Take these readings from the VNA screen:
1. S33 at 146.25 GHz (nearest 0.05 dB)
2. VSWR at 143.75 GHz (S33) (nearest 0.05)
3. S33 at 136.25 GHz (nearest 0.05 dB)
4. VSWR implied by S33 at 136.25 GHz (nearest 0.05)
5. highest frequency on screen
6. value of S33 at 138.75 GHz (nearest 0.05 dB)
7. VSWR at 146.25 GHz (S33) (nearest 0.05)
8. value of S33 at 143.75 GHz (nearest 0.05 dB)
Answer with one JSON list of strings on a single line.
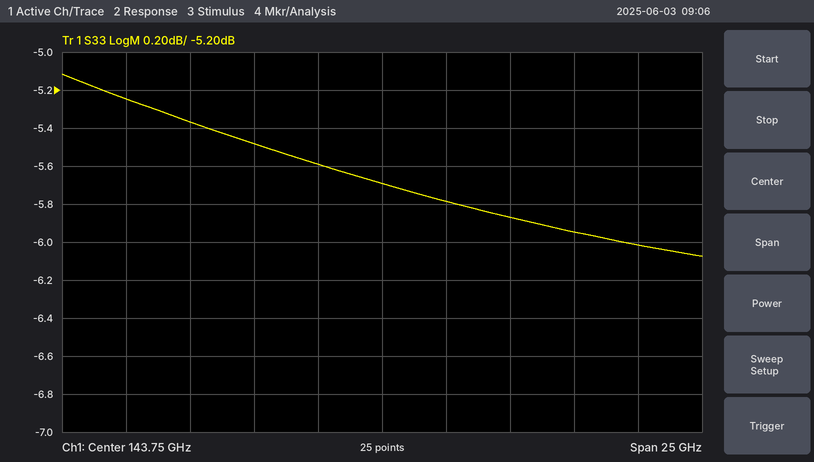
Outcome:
["-5.80 dB", "3.15", "-5.35 dB", "3.35", "156.25 GHz", "-5.50 dB", "3.10", "-5.70 dB"]
